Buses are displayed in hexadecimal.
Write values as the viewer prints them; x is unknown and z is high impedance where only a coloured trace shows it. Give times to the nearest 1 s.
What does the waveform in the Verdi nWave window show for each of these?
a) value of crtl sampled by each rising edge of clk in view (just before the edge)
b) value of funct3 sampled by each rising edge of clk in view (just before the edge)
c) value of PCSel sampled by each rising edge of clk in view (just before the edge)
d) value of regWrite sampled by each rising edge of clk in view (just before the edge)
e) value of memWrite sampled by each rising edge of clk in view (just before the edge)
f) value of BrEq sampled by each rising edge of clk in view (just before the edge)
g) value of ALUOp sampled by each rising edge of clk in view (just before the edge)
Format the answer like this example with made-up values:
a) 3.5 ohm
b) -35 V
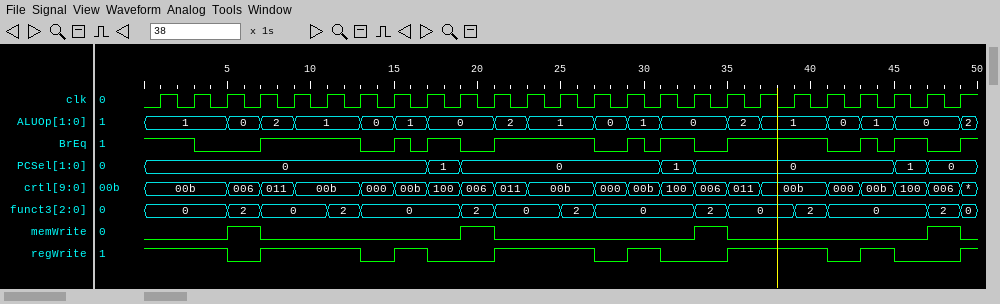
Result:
a) 00b, 00b, 00b, 006, 011, 00b, 00b, 000, 00b, 100, 006, 011, 00b, 00b, 000, 00b, 100, 006, 011, 00b, 00b, 000, 00b, 100, 006
b) 0, 0, 0, 2, 0, 0, 2, 0, 0, 0, 2, 0, 0, 2, 0, 0, 0, 2, 0, 0, 2, 0, 0, 0, 2
c) 0, 0, 0, 0, 0, 0, 0, 0, 0, 1, 0, 0, 0, 0, 0, 0, 1, 0, 0, 0, 0, 0, 0, 1, 0
d) 1 1 1 0 1 1 1 0 1 0 0 1 1 1 0 1 0 0 1 1 1 0 1 0 0
e) 0 0 0 1 0 0 0 0 0 0 1 0 0 0 0 0 0 1 0 0 0 0 0 0 1
f) 1 1 0 0 1 1 1 0 0 1 0 1 1 1 0 0 1 0 1 1 1 0 0 1 0
g) 1, 1, 1, 0, 2, 1, 1, 0, 1, 0, 0, 2, 1, 1, 0, 1, 0, 0, 2, 1, 1, 0, 1, 0, 0
